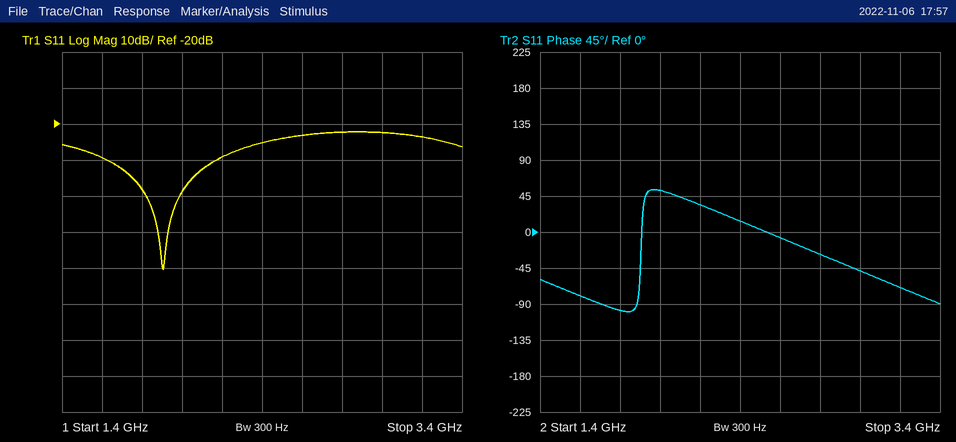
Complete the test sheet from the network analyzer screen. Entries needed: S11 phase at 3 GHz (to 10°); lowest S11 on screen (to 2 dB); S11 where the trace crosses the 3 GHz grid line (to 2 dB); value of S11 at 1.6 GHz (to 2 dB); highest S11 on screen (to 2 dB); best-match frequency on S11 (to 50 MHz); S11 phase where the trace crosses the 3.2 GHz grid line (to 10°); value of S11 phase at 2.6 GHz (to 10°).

-50°
-60 dB
-22 dB
-30 dB
-22 dB
1.90 GHz
-70°
-10°
